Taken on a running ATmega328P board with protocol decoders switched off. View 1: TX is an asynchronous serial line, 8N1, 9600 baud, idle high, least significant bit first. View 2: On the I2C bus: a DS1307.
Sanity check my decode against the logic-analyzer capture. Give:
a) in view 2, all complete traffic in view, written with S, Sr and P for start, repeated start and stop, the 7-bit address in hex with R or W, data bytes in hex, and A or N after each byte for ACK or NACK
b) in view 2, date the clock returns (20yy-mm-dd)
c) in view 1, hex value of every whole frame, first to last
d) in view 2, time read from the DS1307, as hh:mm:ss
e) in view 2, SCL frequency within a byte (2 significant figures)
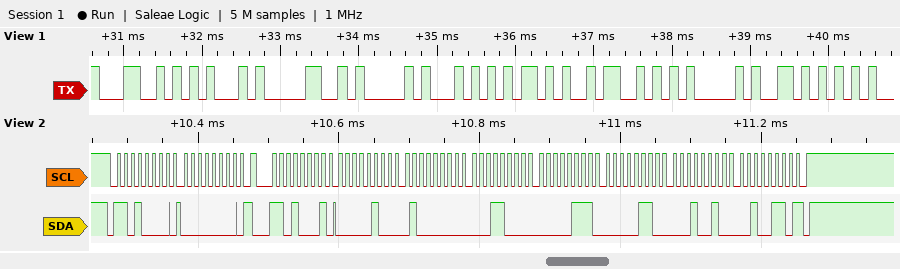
S 68W A 00 A Sr 68R A 04 A 40 A 18 A 07 A 06 A 12 A 26 N P
2026-12-06
4C 45 30 41 54 2B 53 41 56
18:40:04
100 kHz
